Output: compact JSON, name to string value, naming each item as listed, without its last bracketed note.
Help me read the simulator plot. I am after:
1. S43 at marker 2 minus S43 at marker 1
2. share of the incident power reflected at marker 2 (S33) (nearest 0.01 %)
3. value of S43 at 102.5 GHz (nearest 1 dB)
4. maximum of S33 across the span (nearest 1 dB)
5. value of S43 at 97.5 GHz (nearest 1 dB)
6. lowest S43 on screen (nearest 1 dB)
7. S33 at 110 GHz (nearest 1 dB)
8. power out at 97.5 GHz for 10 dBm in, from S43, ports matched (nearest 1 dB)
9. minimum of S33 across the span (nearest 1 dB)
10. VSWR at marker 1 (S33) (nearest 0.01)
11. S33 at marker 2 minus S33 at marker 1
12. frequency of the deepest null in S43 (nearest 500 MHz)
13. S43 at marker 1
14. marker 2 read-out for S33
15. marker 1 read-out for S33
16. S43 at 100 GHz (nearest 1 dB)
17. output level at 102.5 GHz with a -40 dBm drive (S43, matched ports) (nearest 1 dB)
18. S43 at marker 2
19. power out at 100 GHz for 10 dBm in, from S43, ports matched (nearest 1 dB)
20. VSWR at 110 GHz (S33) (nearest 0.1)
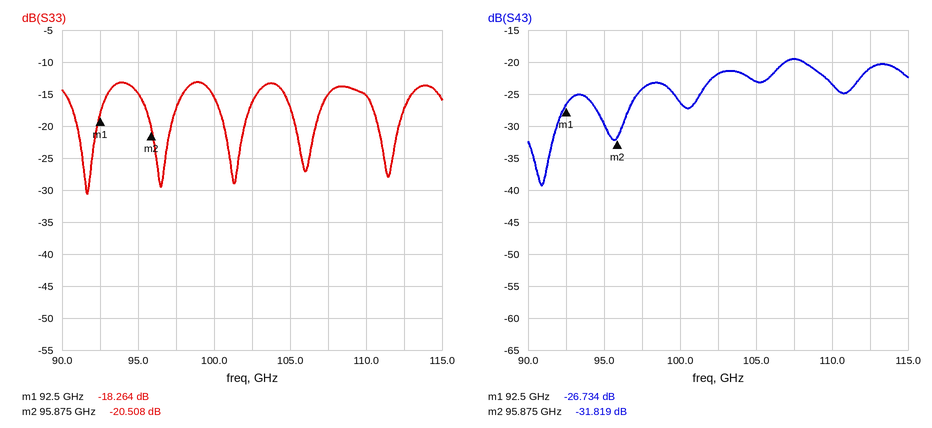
{"S43 at marker 2 minus S43 at marker 1": "-5.085 dB", "share of the incident power reflected at marker 2 (S33)": "0.89 %", "value of S43 at 102.5 GHz": "-22 dB", "maximum of S33 across the span": "-13 dB", "value of S43 at 97.5 GHz": "-24 dB", "lowest S43 on screen": "-39 dB", "S33 at 110 GHz": "-15 dB", "power out at 97.5 GHz for 10 dBm in, from S43, ports matched": "-14 dBm", "minimum of S33 across the span": "-31 dB", "VSWR at marker 1 (S33)": "1.28", "S33 at marker 2 minus S33 at marker 1": "-2.244 dB", "frequency of the deepest null in S43": "91.0 GHz", "S43 at marker 1": "-26.734 dB", "marker 2 read-out for S33": "-20.508 dB", "marker 1 read-out for S33": "-18.264 dB", "S43 at 100 GHz": "-26 dB", "output level at 102.5 GHz with a -40 dBm drive (S43, matched ports)": "-62 dBm", "S43 at marker 2": "-31.819 dB", "power out at 100 GHz for 10 dBm in, from S43, ports matched": "-16 dBm", "VSWR at 110 GHz (S33)": "1.4"}
